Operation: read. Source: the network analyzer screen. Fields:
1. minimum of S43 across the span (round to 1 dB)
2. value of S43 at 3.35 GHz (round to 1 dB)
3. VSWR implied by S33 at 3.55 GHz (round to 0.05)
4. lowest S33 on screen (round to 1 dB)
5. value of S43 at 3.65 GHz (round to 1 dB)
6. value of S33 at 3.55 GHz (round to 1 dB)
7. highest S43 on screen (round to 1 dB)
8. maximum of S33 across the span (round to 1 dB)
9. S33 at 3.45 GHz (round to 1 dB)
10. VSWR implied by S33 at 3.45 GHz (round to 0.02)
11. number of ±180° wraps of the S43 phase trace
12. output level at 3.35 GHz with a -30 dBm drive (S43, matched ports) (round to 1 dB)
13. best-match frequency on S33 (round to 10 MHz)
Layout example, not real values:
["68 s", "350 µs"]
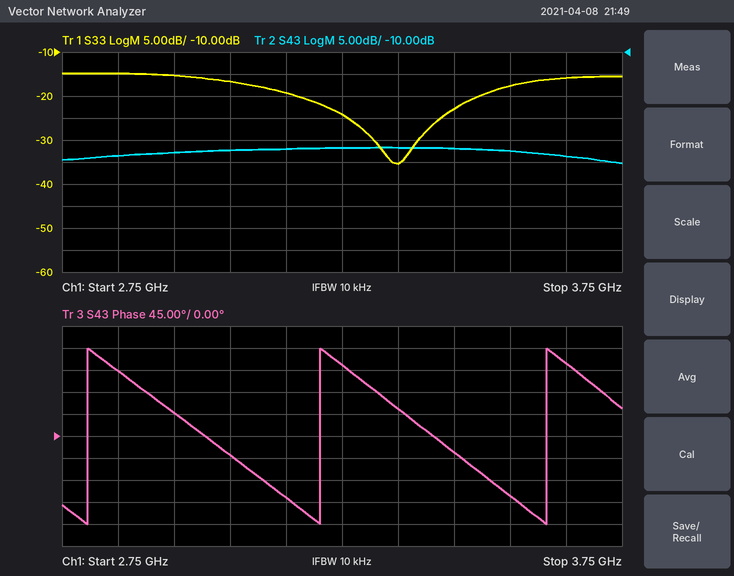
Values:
["-35 dB", "-32 dB", "1.30", "-35 dB", "-34 dB", "-18 dB", "-32 dB", "-15 dB", "-23 dB", "1.16", "3", "-62 dBm", "3.35 GHz"]
